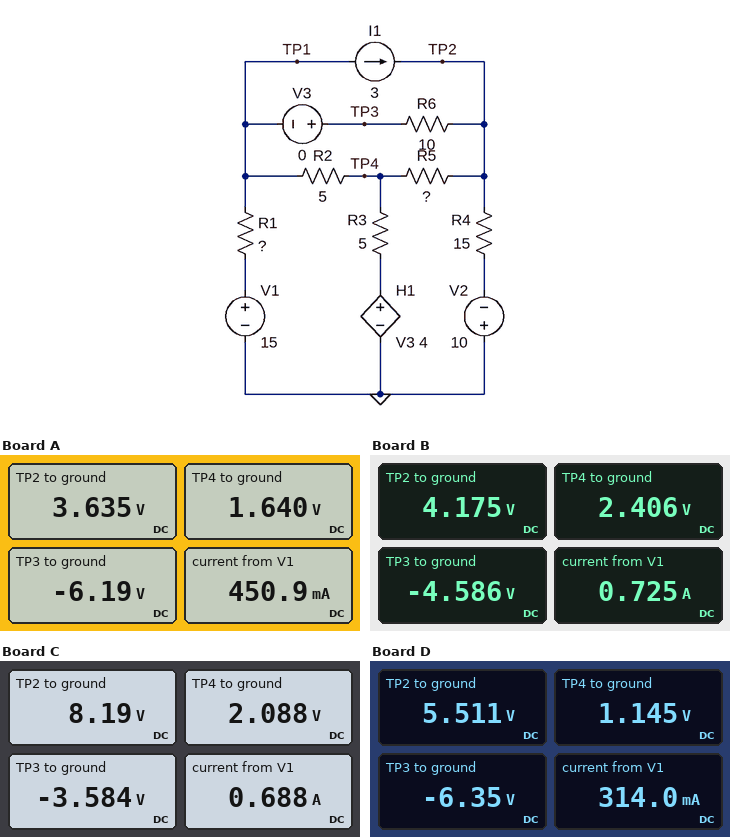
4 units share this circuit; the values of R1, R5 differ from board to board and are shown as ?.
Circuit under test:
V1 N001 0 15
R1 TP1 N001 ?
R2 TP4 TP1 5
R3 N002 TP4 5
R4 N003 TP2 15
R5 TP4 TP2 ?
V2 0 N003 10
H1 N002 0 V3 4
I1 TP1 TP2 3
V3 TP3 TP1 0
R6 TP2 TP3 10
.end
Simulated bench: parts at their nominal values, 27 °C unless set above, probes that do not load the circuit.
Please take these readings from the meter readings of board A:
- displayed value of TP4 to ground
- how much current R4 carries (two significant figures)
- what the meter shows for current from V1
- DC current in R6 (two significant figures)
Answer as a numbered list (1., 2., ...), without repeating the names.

1. 1.640 V
2. 910 mA
3. 450.9 mA
4. 980 mA
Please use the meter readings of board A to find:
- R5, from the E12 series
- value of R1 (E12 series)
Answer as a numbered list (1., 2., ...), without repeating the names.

1. 1.8 Ω
2. 47 Ω
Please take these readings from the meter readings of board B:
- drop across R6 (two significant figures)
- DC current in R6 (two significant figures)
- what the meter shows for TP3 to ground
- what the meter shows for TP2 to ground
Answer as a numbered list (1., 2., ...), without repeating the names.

1. 8.8 V
2. 880 mA
3. -4.586 V
4. 4.175 V
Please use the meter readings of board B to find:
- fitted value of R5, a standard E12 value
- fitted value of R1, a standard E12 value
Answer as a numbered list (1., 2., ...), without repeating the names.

1. 1.5 Ω
2. 27 Ω
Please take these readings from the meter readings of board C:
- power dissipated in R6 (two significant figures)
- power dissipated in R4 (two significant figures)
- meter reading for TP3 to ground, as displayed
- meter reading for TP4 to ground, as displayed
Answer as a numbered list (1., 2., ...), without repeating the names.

1. 14 W
2. 22 W
3. -3.584 V
4. 2.088 V
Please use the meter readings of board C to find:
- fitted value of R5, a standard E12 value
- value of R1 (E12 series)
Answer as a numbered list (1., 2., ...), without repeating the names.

1. 10 Ω
2. 27 Ω
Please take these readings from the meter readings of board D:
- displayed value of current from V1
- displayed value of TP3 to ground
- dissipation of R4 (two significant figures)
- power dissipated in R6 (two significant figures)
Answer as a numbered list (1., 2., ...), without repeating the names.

1. 314.0 mA
2. -6.35 V
3. 16 W
4. 14 W
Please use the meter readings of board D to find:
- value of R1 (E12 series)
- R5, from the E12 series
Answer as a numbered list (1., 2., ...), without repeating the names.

1. 68 Ω
2. 5.6 Ω
